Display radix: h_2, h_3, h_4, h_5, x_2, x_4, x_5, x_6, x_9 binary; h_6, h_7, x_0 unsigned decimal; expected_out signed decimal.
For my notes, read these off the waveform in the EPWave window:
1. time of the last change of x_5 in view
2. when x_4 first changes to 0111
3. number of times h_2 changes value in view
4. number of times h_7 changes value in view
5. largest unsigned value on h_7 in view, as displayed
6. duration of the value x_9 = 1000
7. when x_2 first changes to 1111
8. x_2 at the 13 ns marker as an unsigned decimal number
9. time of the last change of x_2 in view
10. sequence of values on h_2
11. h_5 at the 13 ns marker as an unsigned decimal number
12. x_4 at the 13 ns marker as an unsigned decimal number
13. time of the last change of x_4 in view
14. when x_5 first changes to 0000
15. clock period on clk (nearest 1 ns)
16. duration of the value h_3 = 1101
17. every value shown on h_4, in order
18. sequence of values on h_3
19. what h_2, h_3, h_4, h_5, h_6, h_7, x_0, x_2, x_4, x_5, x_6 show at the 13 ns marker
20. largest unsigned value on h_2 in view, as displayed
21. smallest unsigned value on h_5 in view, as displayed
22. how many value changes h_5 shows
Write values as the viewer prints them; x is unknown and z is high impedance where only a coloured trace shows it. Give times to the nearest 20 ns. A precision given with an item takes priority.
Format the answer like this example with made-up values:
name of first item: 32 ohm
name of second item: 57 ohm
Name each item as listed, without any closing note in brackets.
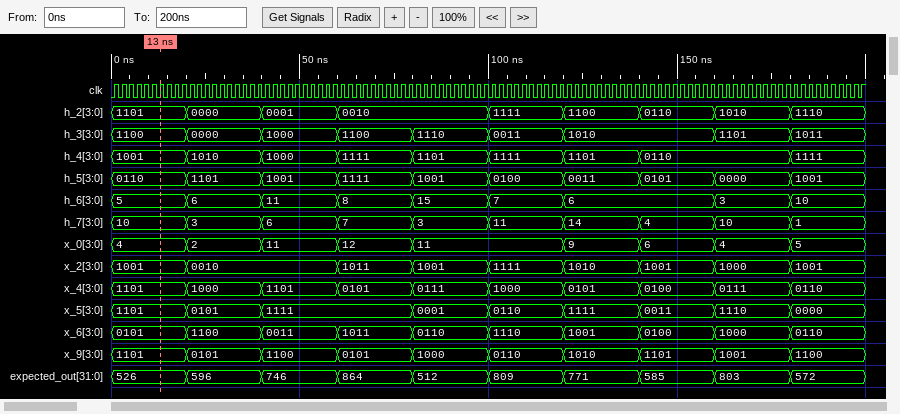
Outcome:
time of the last change of x_5 in view: 180 ns
when x_4 first changes to 0111: 80 ns
number of times h_2 changes value in view: 8
number of times h_7 changes value in view: 9
largest unsigned value on h_7 in view, as displayed: 14
duration of the value x_9 = 1000: 20 ns
when x_2 first changes to 1111: 100 ns
x_2 at the 13 ns marker as an unsigned decimal number: 9
time of the last change of x_2 in view: 180 ns
sequence of values on h_2: 1101, 0000, 0001, 0010, 1111, 1100, 0110, 1010, 1110
h_5 at the 13 ns marker as an unsigned decimal number: 6
x_4 at the 13 ns marker as an unsigned decimal number: 13
time of the last change of x_4 in view: 180 ns
when x_5 first changes to 0000: 180 ns
clock period on clk: 2 ns
duration of the value h_3 = 1101: 20 ns
every value shown on h_4, in order: 1001, 1010, 1000, 1111, 1101, 1111, 1101, 0110, 1111
sequence of values on h_3: 1100, 0000, 1000, 1100, 1110, 0011, 1010, 1101, 1011
what h_2, h_3, h_4, h_5, h_6, h_7, x_0, x_2, x_4, x_5, x_6 show at the 13 ns marker: h_2=1101, h_3=1100, h_4=1001, h_5=0110, h_6=5, h_7=10, x_0=4, x_2=1001, x_4=1101, x_5=1101, x_6=0101
largest unsigned value on h_2 in view, as displayed: 1111
smallest unsigned value on h_5 in view, as displayed: 0000
how many value changes h_5 shows: 9
